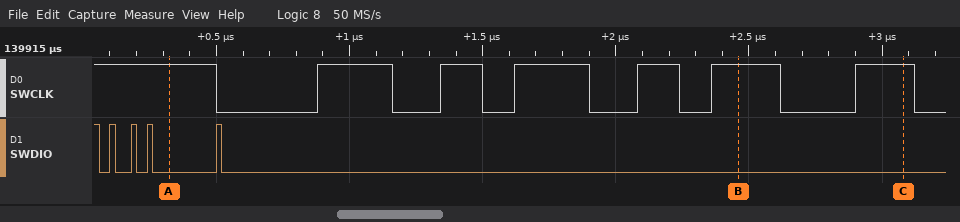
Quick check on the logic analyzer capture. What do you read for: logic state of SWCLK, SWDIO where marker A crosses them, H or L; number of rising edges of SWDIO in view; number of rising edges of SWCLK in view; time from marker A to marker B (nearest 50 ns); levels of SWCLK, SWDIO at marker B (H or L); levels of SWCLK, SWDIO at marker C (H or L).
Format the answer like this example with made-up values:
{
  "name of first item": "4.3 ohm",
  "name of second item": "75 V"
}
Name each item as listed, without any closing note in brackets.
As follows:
{
  "logic state of SWCLK, SWDIO where marker A crosses them, H or L": "SWCLK=H, SWDIO=L",
  "number of rising edges of SWDIO in view": "4",
  "number of rising edges of SWCLK in view": "6",
  "time from marker A to marker B": "2150 ns",
  "levels of SWCLK, SWDIO at marker B": "SWCLK=H, SWDIO=L",
  "levels of SWCLK, SWDIO at marker C": "SWCLK=H, SWDIO=L"
}
